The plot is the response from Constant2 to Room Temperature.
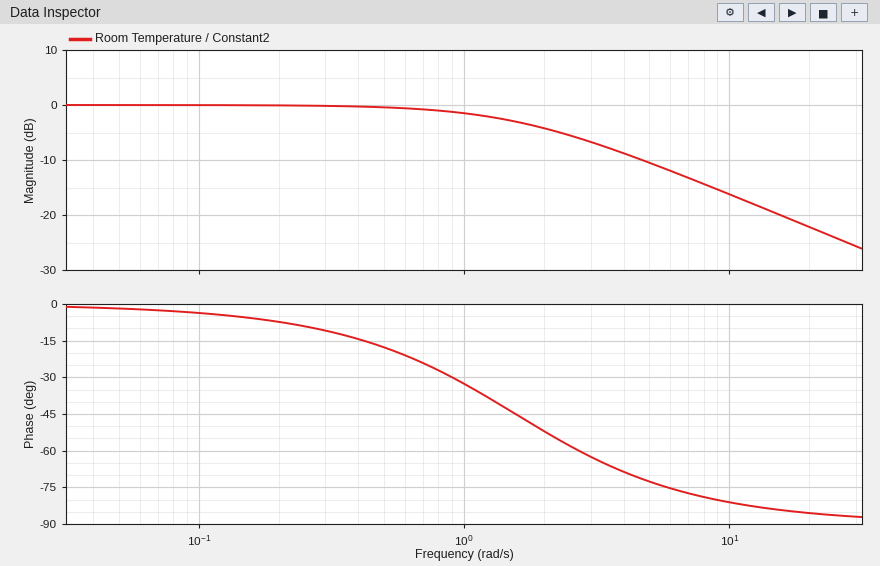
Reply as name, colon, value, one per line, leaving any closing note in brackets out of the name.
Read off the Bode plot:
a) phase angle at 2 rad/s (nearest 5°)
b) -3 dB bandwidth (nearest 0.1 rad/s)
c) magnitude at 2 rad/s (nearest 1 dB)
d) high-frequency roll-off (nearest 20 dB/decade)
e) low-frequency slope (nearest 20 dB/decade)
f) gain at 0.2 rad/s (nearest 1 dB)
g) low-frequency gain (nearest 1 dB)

phase angle at 2 rad/s: -50°
-3 dB bandwidth: 1.6 rad/s
magnitude at 2 rad/s: -4 dB
high-frequency roll-off: -20 dB/decade
low-frequency slope: 0 dB/decade
gain at 0.2 rad/s: 0 dB
low-frequency gain: 0 dB
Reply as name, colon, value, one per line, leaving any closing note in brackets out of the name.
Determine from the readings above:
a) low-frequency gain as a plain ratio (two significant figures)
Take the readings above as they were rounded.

low-frequency gain as a plain ratio: 1.0
